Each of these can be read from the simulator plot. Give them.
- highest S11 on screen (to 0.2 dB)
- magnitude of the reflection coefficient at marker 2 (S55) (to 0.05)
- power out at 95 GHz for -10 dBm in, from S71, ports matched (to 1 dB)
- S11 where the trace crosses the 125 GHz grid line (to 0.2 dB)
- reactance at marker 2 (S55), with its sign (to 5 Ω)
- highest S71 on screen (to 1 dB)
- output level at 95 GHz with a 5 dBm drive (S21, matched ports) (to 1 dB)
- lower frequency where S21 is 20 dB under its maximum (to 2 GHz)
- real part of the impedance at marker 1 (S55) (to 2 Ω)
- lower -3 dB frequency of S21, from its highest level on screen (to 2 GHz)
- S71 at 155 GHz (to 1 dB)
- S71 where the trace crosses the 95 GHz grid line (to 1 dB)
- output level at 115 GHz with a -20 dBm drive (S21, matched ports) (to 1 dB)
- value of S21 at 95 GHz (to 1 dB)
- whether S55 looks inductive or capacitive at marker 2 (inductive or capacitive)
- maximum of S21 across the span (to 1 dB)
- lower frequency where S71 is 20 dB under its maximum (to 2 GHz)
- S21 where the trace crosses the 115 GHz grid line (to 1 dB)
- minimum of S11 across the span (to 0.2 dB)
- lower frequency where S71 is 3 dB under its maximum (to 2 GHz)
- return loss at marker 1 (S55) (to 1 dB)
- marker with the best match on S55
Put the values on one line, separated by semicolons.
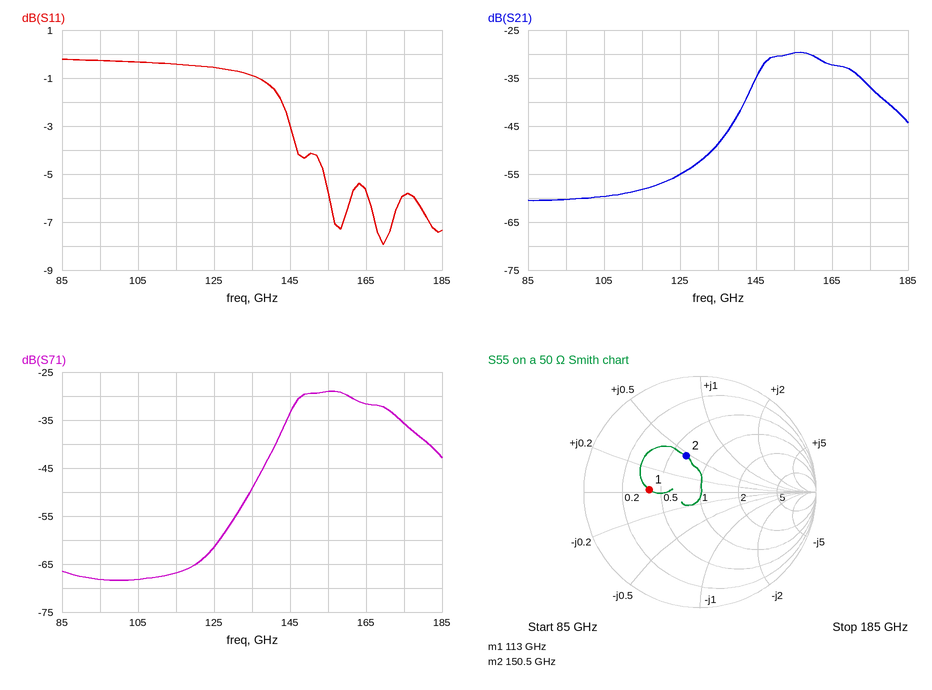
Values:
-0.2 dB; 0.35; -78 dBm; -0.6 dB; +25 Ω; -29 dB; -55 dBm; 134 GHz; 20 Ω; 146 GHz; -29 dB; -68 dB; -78 dBm; -60 dB; inductive; -30 dB; 136 GHz; -58 dB; -8.0 dB; 146 GHz; 7 dB; marker 2
